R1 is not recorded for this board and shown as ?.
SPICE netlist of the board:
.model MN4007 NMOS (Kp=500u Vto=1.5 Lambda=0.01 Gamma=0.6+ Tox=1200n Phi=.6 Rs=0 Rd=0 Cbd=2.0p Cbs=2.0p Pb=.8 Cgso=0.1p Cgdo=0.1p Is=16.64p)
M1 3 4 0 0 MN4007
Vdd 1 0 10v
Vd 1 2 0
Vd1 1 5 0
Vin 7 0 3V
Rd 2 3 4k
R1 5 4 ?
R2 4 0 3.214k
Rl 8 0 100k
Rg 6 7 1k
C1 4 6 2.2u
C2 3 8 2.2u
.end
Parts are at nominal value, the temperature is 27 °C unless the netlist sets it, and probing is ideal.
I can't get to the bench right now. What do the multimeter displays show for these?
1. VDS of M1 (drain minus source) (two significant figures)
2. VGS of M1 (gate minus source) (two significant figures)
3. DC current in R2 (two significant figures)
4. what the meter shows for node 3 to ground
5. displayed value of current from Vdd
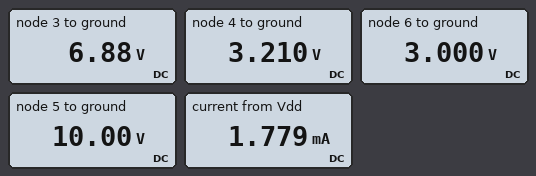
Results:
6.9 V
3.2 V
1.0 mA
6.88 V
1.779 mA
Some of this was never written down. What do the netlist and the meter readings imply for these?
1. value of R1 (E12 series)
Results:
6.8 kΩ
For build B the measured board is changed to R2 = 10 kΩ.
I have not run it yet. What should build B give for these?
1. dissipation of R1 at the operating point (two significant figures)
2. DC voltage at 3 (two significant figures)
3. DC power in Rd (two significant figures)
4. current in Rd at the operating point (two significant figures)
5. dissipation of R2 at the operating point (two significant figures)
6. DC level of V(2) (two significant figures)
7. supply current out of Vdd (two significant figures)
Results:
2.4 mW
1.1 V
20 mW
2.2 mA
3.5 mW
10 V
2.8 mA
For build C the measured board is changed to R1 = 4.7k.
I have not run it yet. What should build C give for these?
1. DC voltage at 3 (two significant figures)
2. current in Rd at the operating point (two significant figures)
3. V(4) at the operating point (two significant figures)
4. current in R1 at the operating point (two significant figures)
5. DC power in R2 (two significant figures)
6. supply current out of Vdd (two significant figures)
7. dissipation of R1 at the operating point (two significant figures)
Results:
3.2 V
1.7 mA
4.1 V
1.3 mA
5.1 mW
3.0 mA
7.5 mW
